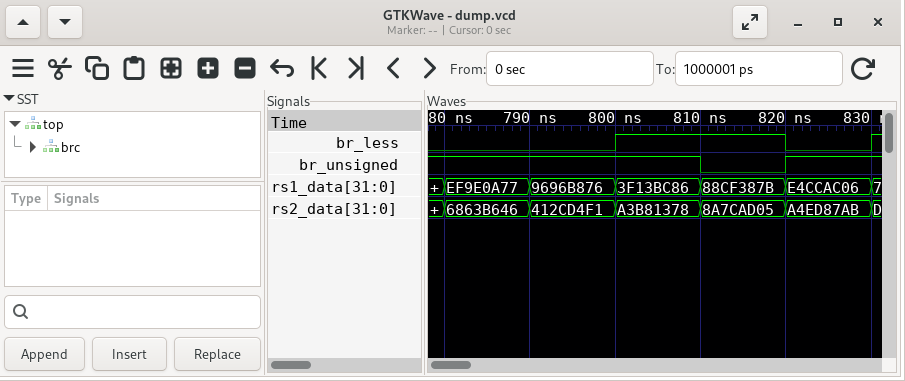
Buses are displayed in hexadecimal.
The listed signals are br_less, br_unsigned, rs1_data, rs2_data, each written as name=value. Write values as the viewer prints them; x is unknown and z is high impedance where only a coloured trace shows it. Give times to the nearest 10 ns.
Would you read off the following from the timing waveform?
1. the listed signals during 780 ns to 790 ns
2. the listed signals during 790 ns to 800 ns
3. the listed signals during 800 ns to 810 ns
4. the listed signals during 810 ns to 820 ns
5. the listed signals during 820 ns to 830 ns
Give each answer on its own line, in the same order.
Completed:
br_less=0, br_unsigned=1, rs1_data=EF9E0A77, rs2_data=6863B646
br_less=0, br_unsigned=1, rs1_data=9696B876, rs2_data=412CD4F1
br_less=1, br_unsigned=1, rs1_data=3F13BC86, rs2_data=A3B81378
br_less=1, br_unsigned=0, rs1_data=88CF387B, rs2_data=8A7CAD05
br_less=0, br_unsigned=1, rs1_data=E4CCAC06, rs2_data=A4ED87AB
